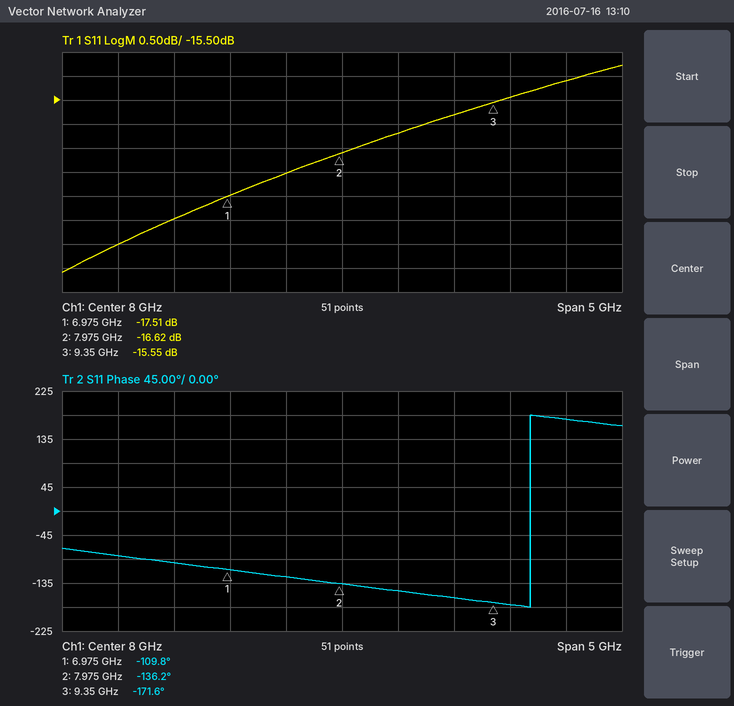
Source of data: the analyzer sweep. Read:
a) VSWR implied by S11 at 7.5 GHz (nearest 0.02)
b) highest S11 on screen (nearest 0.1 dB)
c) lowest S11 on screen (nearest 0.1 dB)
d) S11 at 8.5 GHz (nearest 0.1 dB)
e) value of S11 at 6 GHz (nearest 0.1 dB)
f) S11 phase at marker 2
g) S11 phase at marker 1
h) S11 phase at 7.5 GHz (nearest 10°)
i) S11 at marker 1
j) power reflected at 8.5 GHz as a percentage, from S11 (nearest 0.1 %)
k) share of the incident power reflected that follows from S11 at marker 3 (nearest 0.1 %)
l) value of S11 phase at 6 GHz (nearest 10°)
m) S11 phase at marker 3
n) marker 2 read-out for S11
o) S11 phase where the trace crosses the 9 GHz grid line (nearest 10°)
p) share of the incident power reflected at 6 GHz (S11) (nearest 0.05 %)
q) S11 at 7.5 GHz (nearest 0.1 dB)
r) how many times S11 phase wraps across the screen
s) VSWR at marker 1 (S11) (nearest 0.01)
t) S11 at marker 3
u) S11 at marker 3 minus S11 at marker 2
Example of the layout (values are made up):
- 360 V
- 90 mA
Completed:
- 1.32
- -14.8 dB
- -19.1 dB
- -16.2 dB
- -18.5 dB
- -136.2°
- -109.8°
- -120°
- -17.51 dB
- 2.4 %
- 2.8 %
- -80°
- -171.6°
- -16.62 dB
- -160°
- 1.40 %
- -17.0 dB
- 1
- 1.31
- -15.55 dB
- 1.07 dB
